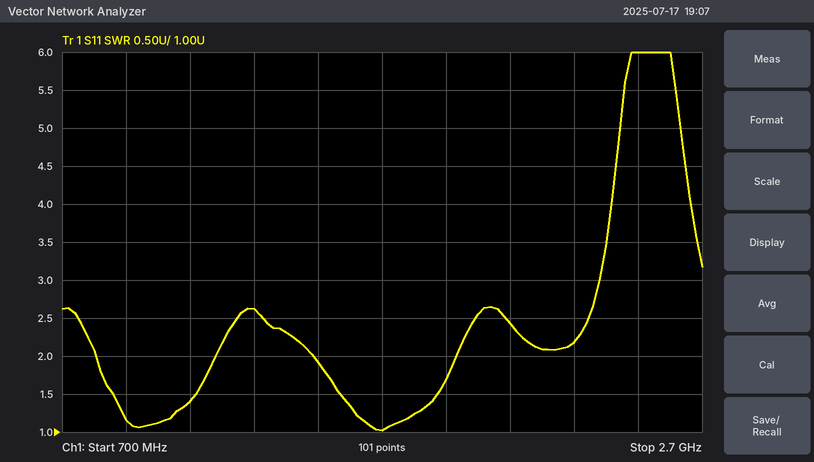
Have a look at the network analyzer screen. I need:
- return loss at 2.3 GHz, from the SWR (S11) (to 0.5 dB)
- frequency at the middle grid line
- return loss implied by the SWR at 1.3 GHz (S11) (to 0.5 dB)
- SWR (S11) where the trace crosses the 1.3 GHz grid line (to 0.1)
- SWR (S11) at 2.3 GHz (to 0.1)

8.5 dB
1.7 GHz
7.0 dB
2.6
2.2
